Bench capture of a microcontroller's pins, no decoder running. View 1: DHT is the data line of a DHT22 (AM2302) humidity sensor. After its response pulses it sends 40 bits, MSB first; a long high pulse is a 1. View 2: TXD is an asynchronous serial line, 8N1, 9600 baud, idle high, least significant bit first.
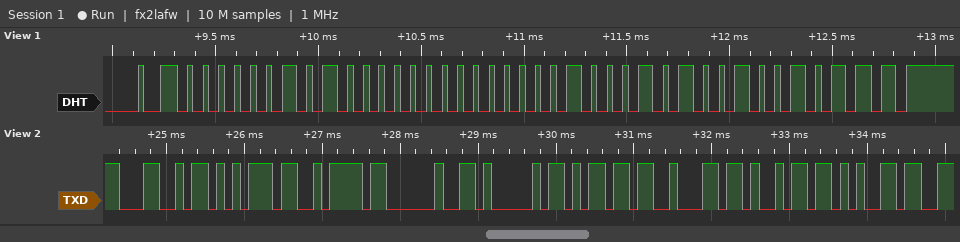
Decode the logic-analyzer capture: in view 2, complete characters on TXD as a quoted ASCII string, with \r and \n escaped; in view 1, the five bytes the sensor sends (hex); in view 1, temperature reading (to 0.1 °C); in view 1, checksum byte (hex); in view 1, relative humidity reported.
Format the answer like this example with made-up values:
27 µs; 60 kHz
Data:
"Luz Ambie"; 02 80 01 14 97; 27.6 °C; 0x97; 64.0 %
